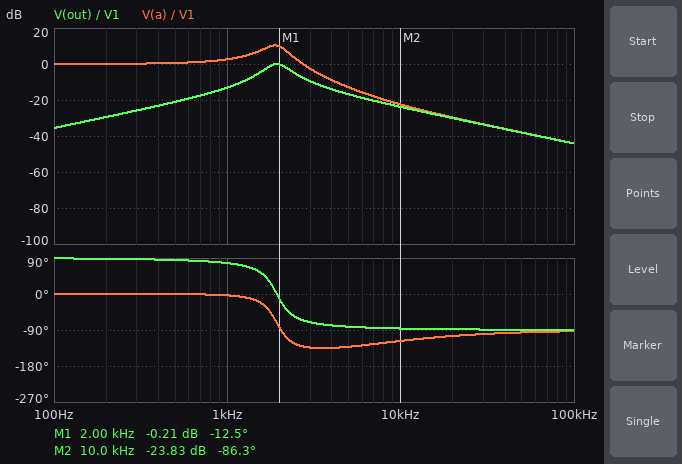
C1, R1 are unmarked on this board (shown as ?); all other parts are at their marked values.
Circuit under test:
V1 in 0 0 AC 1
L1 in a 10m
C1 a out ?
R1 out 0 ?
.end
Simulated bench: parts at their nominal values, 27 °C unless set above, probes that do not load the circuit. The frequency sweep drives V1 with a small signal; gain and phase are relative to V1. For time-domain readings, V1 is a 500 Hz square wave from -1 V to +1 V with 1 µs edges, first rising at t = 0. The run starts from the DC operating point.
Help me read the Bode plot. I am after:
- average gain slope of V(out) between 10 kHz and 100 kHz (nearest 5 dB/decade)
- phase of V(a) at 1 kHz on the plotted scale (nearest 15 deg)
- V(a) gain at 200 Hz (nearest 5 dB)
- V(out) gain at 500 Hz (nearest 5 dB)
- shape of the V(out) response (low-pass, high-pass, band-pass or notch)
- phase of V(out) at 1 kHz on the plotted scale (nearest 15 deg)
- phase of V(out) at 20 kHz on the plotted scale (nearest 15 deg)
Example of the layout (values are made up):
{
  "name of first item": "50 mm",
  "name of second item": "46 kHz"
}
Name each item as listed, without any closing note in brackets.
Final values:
{
  "average gain slope of V(out) between 10 kHz and 100 kHz": "-20 dB/decade",
  "phase of V(a) at 1 kHz on the plotted scale": "0 deg",
  "V(a) gain at 200 Hz": "0 dB",
  "V(out) gain at 500 Hz": "-20 dB",
  "shape of the V(out) response": "band-pass",
  "phase of V(out) at 1 kHz on the plotted scale": "75 deg",
  "phase of V(out) at 20 kHz on the plotted scale": "-90 deg"
}
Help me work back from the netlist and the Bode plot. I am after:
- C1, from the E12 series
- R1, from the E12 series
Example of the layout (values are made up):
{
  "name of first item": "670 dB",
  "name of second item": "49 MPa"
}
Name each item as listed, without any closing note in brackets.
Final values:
{
  "C1, from the E12 series": "680 nF",
  "R1, from the E12 series": "39 Ω"
}
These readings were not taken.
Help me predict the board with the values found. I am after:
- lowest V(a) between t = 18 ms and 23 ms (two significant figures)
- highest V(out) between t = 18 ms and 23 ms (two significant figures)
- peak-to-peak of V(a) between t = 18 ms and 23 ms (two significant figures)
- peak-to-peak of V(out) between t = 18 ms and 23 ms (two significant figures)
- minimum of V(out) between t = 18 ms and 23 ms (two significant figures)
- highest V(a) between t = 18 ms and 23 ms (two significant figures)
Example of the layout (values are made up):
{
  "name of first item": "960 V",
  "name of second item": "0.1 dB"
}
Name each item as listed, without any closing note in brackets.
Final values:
{
  "lowest V(a) between t = 18 ms and 23 ms": "-2.1 V",
  "highest V(out) between t = 18 ms and 23 ms": "460 mV",
  "peak-to-peak of V(a) between t = 18 ms and 23 ms": "4.3 V",
  "peak-to-peak of V(out) between t = 18 ms and 23 ms": "920 mV",
  "minimum of V(out) between t = 18 ms and 23 ms": "-460 mV",
  "highest V(a) between t = 18 ms and 23 ms": "2.1 V"
}
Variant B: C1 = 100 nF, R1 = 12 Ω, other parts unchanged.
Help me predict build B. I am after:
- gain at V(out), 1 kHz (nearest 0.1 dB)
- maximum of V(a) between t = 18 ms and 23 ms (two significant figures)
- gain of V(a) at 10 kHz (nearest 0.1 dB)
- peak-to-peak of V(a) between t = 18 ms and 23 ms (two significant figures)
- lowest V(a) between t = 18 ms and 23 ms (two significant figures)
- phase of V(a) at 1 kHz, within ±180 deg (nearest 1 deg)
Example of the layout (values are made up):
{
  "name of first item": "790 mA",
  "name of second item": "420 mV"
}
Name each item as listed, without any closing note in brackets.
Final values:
{
  "gain at V(out), 1 kHz": "-42.1 dB",
  "maximum of V(a) between t = 18 ms and 23 ms": "2.2 V",
  "gain of V(a) at 10 kHz": "-9.4 dB",
  "peak-to-peak of V(a) between t = 18 ms and 23 ms": "4.4 V",
  "lowest V(a) between t = 18 ms and 23 ms": "-2.2 V",
  "phase of V(a) at 1 kHz, within ±180 deg": "0 deg"
}
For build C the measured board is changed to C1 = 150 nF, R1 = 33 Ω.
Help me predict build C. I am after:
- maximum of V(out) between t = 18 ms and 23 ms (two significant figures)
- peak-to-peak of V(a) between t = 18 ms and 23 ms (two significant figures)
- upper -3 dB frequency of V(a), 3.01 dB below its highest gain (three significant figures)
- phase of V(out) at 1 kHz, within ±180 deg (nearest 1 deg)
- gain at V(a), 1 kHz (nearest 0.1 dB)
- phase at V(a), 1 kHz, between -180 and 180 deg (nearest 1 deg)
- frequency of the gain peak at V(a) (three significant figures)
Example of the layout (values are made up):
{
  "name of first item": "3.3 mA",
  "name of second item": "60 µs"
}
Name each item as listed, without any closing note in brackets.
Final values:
{
  "maximum of V(out) between t = 18 ms and 23 ms": "200 mV",
  "peak-to-peak of V(a) between t = 18 ms and 23 ms": "4.8 V",
  "upper -3 dB frequency of V(a), 3.01 dB below its highest gain": "4.35 kHz",
  "phase of V(out) at 1 kHz, within ±180 deg": "88 deg",
  "gain at V(a), 1 kHz": "0.5 dB",
  "phase at V(a), 1 kHz, between -180 and 180 deg": "0 deg",
  "frequency of the gain peak at V(a)": "4.09 kHz"
}
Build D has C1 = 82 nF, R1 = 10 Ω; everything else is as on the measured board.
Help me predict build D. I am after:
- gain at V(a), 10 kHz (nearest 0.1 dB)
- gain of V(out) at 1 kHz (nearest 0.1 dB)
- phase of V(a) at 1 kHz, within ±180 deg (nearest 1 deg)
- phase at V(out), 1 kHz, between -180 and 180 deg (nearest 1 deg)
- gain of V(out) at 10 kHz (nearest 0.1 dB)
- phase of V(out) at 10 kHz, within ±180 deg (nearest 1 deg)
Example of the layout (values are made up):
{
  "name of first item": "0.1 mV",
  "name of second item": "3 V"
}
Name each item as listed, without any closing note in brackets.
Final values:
{
  "gain at V(a), 10 kHz": "-7.0 dB",
  "gain of V(out) at 1 kHz": "-45.5 dB",
  "phase of V(a) at 1 kHz, within ±180 deg": "0 deg",
  "phase at V(out), 1 kHz, between -180 and 180 deg": "90 deg",
  "gain of V(out) at 10 kHz": "-32.8 dB",
  "phase of V(out) at 10 kHz, within ±180 deg": "-89 deg"
}
